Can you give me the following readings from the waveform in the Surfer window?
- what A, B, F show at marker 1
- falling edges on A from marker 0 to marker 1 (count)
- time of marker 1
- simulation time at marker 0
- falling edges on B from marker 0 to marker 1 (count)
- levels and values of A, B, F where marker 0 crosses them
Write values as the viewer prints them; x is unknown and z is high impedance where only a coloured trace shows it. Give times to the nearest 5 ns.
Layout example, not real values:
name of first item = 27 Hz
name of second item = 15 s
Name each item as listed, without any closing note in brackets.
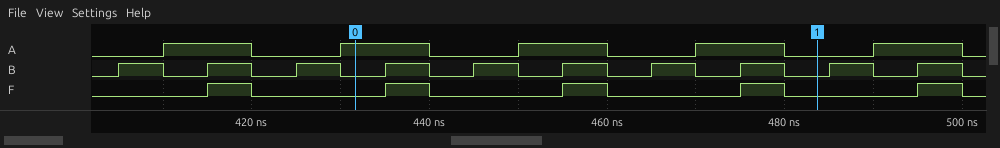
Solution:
what A, B, F show at marker 1 = A=0, B=0, F=0
falling edges on A from marker 0 to marker 1 = 3
time of marker 1 = 485 ns
simulation time at marker 0 = 430 ns
falling edges on B from marker 0 to marker 1 = 5
levels and values of A, B, F where marker 0 crosses them = A=1, B=0, F=0
